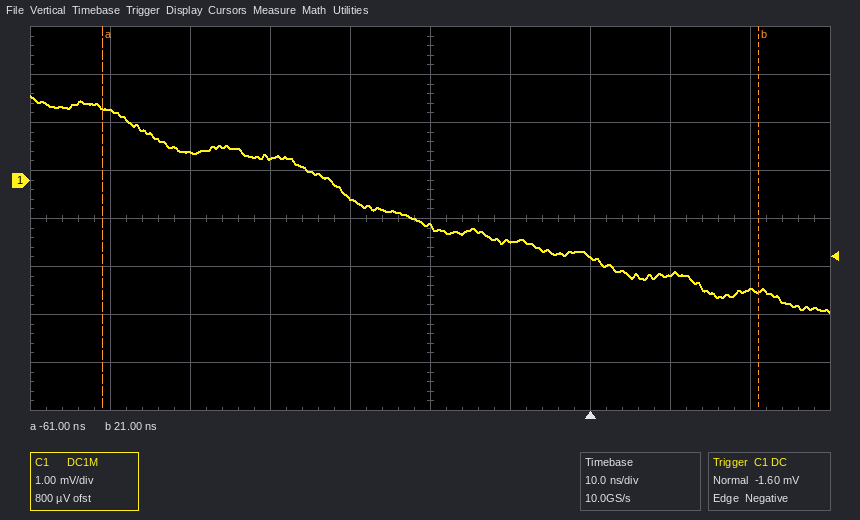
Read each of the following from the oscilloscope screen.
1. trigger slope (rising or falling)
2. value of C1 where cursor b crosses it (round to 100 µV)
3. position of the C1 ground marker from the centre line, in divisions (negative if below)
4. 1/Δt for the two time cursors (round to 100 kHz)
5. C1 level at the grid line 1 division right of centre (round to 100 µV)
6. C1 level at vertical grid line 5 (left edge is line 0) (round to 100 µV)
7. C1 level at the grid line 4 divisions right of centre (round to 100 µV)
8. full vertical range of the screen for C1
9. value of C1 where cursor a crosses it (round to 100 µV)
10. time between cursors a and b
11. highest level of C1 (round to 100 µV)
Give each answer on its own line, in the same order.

falling
-2.3 mV
+0.8 div
12.2 MHz
-1.3 mV
-1.0 mV
-2.3 mV
8 mV
1.5 mV
82 ns
1.8 mV
